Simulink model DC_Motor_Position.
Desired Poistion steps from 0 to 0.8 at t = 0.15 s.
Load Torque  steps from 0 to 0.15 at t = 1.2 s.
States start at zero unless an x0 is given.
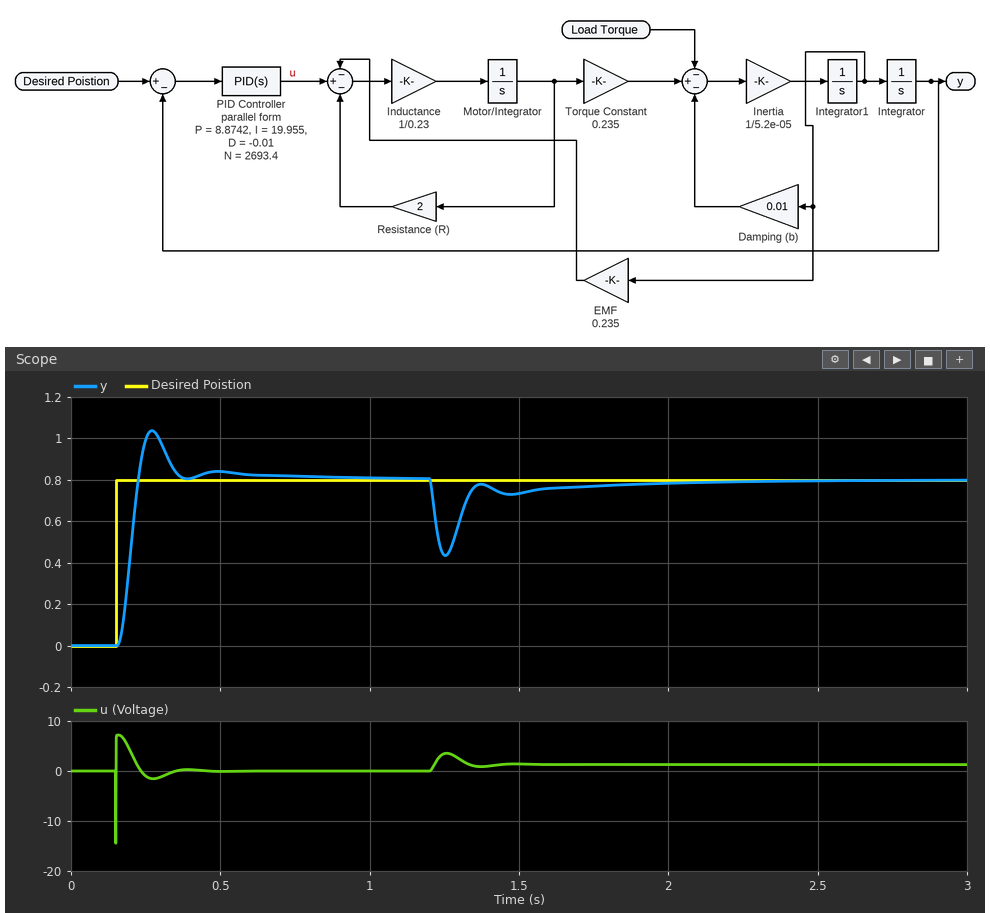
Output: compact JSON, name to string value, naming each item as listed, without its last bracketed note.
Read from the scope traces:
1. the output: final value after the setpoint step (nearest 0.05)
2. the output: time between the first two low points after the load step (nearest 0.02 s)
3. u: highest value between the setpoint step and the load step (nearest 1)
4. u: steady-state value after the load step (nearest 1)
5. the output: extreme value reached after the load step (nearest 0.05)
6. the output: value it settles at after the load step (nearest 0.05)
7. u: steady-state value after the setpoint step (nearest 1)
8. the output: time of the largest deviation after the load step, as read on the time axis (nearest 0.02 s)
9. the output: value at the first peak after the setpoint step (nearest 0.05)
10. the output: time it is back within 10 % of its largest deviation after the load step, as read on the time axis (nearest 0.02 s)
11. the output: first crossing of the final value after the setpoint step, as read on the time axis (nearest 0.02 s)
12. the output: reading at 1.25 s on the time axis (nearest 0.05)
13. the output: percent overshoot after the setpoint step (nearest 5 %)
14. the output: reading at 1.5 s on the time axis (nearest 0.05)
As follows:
{"the output: final value after the setpoint step": "0.80", "the output: time between the first two low points after the load step": "0.22 s", "u: highest value between the setpoint step and the load step": "7", "u: steady-state value after the load step": "1", "the output: extreme value reached after the load step": "0.45", "the output: value it settles at after the load step": "0.80", "u: steady-state value after the setpoint step": "0", "the output: time of the largest deviation after the load step, as read on the time axis": "1.26 s", "the output: value at the first peak after the setpoint step": "1.05", "the output: time it is back within 10 % of its largest deviation after the load step, as read on the time axis": "1.66 s", "the output: first crossing of the final value after the setpoint step, as read on the time axis": "0.22 s", "the output: reading at 1.25 s on the time axis": "0.45", "the output: percent overshoot after the setpoint step": "30 %", "the output: reading at 1.5 s on the time axis": "0.75"}
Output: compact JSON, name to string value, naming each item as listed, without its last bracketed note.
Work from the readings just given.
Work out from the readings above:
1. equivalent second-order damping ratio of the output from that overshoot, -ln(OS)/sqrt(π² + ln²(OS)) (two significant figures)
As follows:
{"equivalent second-order damping ratio of the output from that overshoot, -ln(OS)/sqrt(π² + ln²(OS))": "0.36"}
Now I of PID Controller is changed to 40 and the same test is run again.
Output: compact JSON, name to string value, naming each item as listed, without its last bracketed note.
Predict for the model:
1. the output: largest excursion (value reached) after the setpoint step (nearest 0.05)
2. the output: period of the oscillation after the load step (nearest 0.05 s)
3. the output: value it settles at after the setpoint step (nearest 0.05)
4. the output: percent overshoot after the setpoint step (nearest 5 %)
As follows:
{"the output: largest excursion (value reached) after the setpoint step": "1.10", "the output: period of the oscillation after the load step": "0.25 s", "the output: value it settles at after the setpoint step": "0.80", "the output: percent overshoot after the setpoint step": "40 %"}
